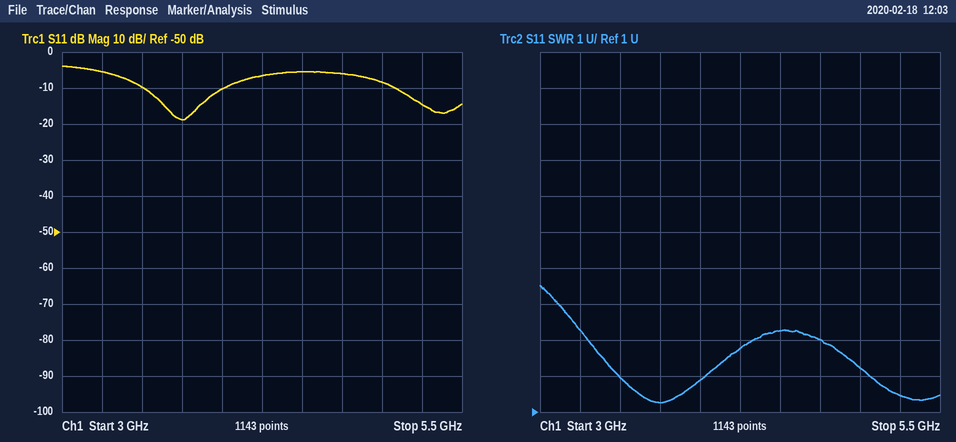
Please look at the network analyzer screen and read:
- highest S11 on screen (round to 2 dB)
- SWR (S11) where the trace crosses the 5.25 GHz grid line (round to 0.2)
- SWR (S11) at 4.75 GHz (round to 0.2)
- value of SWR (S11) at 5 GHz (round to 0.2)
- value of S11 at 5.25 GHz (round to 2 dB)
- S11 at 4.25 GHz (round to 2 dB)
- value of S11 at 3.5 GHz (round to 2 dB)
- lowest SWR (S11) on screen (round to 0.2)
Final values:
-4 dB
1.4
3.0
2.2
-14 dB
-6 dB
-10 dB
1.2
